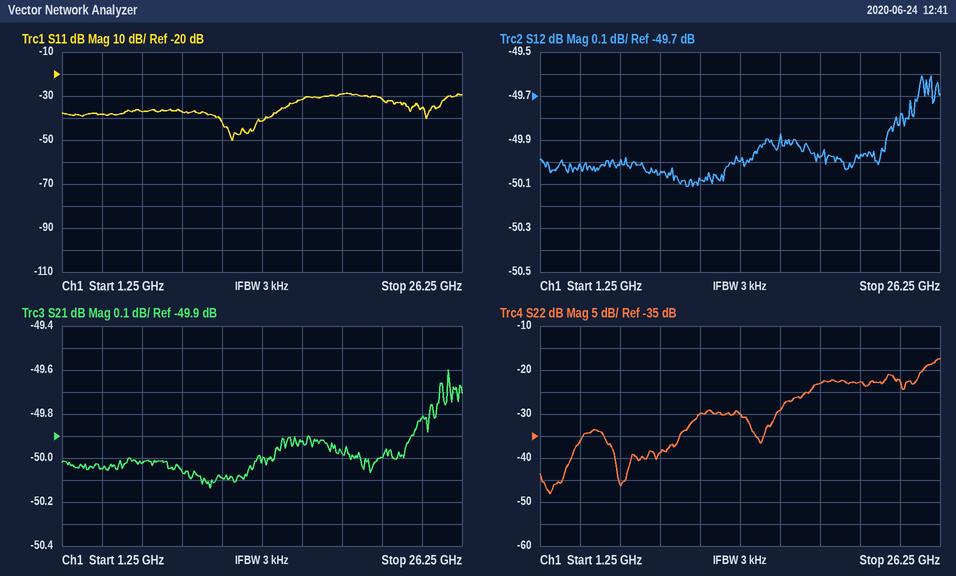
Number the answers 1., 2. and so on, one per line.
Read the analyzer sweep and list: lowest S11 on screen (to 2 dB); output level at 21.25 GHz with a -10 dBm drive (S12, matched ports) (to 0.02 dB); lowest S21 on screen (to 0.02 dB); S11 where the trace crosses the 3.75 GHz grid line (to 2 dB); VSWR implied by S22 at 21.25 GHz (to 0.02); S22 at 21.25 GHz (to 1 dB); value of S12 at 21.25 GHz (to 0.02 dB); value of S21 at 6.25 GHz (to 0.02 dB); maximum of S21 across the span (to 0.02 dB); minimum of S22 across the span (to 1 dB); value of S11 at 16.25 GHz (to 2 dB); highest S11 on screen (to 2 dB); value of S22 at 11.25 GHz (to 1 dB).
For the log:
1. -50 dB
2. -59.98 dBm
3. -50.14 dB
4. -38 dB
5. 1.16
6. -23 dB
7. -49.98 dB
8. -50.02 dB
9. -49.60 dB
10. -48 dB
11. -32 dB
12. -28 dB
13. -30 dB
